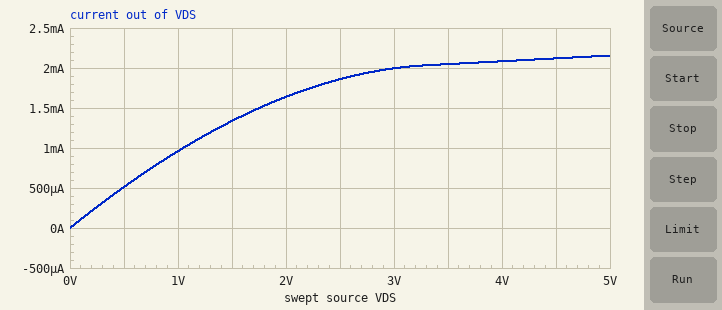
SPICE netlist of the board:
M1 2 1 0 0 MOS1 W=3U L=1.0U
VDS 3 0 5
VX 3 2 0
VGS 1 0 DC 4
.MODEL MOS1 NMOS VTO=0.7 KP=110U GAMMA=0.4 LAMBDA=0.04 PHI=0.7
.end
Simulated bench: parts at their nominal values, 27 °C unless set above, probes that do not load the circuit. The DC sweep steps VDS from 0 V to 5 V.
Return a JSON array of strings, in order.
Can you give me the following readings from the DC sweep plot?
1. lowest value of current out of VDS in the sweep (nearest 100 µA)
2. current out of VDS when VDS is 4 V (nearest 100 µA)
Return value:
["0 A", "2.1 mA"]
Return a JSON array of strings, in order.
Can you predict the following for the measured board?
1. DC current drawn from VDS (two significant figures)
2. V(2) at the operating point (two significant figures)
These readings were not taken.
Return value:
["2.2 mA", "5.0 V"]
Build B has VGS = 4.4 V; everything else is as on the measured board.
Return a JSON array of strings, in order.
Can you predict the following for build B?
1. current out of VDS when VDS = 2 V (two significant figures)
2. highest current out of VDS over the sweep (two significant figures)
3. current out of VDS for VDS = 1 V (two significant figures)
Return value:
["1.9 mA", "2.7 mA", "1.1 mA"]
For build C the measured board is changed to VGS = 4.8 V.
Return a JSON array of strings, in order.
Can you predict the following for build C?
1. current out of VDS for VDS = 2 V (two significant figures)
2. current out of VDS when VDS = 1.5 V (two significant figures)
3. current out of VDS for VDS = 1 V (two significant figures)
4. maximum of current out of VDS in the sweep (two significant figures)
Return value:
["2.2 mA", "1.8 mA", "1.2 mA", "3.3 mA"]
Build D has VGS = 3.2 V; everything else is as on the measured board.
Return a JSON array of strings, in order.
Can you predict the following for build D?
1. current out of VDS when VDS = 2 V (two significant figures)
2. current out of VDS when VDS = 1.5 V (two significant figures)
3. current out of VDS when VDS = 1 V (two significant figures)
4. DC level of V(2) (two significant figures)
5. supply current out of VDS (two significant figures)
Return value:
["1.1 mA", "920 µA", "690 µA", "5.0 V", "1.2 mA"]
